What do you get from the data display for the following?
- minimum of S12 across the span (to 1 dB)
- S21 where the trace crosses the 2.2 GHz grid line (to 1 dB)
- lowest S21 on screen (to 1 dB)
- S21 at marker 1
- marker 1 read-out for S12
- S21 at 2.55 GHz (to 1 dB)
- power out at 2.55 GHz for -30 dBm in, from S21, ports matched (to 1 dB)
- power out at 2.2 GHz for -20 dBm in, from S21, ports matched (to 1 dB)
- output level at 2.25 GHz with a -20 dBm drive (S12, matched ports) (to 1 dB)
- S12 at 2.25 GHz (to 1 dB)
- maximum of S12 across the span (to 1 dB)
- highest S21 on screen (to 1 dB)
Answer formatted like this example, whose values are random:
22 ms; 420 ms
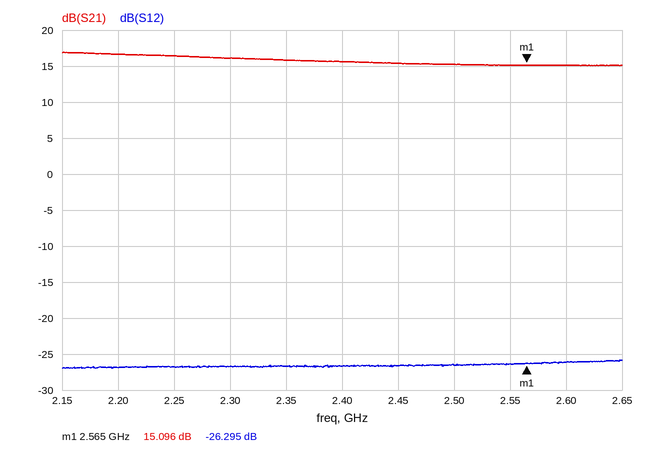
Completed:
-27 dB; 17 dB; 15 dB; 15.096 dB; -26.295 dB; 15 dB; -15 dBm; -3 dBm; -47 dBm; -27 dB; -26 dB; 17 dB
